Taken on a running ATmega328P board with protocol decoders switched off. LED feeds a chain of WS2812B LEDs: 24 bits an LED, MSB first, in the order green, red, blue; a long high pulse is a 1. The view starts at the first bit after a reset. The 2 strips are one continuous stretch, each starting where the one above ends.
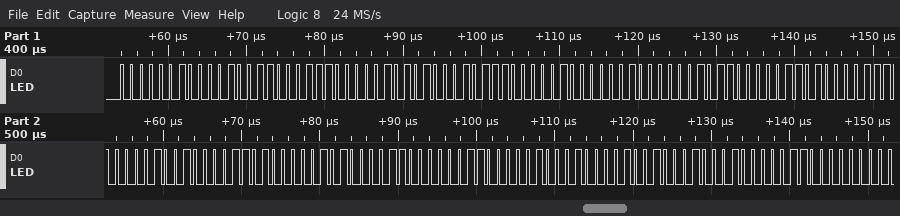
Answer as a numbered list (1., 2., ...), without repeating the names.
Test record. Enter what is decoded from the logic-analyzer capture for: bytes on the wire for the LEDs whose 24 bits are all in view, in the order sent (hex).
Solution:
1. 02 13 1C 15 17 04 08 16 0D 0E 09 0D 05 0C 0C 11 09 11
